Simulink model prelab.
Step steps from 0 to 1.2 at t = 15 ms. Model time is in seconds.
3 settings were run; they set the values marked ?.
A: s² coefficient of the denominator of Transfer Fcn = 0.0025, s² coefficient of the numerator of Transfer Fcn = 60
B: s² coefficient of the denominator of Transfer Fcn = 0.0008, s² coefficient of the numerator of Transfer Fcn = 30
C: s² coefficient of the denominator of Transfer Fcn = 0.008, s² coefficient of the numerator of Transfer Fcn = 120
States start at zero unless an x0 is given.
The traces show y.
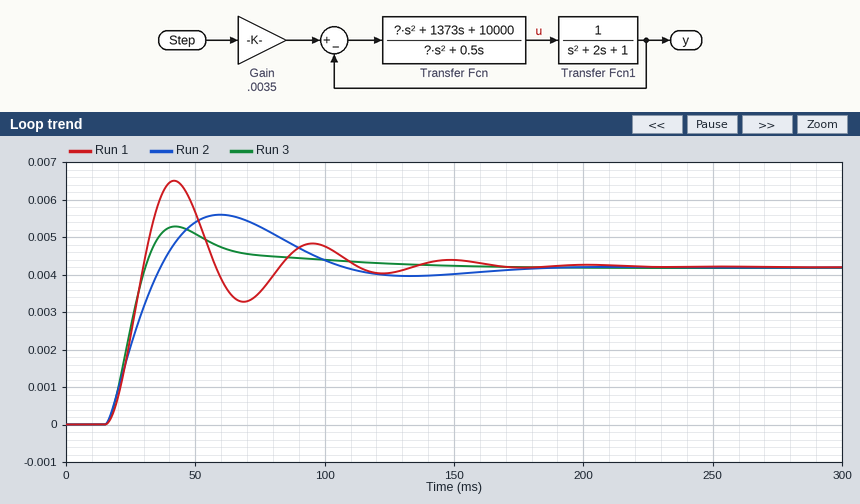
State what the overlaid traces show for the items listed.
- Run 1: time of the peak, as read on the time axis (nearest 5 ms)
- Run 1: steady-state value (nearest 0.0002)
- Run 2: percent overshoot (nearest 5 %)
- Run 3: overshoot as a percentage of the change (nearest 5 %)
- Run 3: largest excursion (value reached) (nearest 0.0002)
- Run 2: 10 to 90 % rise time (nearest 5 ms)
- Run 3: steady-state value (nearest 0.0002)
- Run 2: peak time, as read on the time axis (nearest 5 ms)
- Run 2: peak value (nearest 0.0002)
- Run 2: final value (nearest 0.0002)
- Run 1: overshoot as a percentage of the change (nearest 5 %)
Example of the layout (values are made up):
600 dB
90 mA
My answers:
40 ms
0.0042
35 %
25 %
0.0052
15 ms
0.0042
60 ms
0.0056
0.0042
55 %
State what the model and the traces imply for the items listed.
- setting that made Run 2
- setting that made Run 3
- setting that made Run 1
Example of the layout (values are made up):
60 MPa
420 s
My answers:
B
A
C
